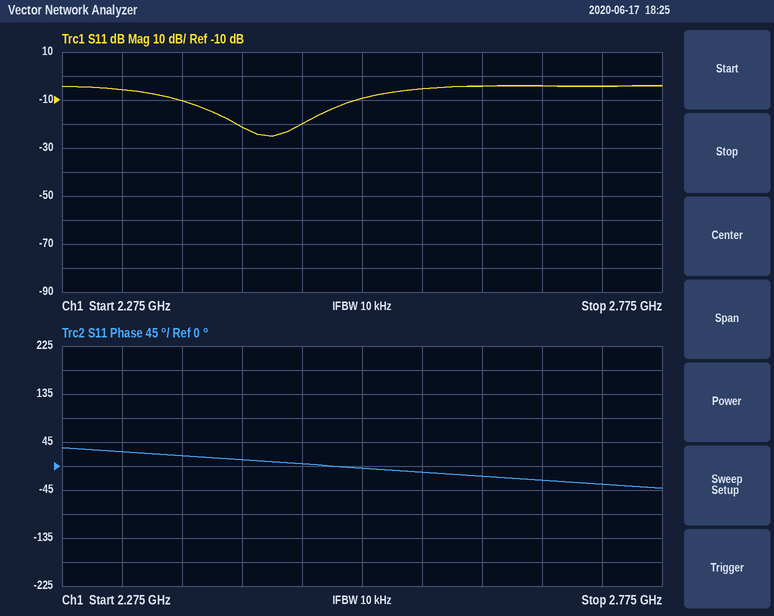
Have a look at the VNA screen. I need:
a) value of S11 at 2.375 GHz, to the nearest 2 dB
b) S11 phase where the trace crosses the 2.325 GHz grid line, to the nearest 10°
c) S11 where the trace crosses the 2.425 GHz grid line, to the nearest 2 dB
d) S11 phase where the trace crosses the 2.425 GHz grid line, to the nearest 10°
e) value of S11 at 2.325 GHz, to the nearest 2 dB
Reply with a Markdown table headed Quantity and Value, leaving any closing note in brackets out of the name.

| Quantity | Value |
|---|---|
| value of S11 at 2.375 GHz, to the nearest 2 dB | -10 dB |
| S11 phase where the trace crosses the 2.325 GHz grid line, to the nearest 10° | 30° |
| S11 where the trace crosses the 2.425 GHz grid line, to the nearest 2 dB | -22 dB |
| S11 phase where the trace crosses the 2.425 GHz grid line, to the nearest 10° | 10° |
| value of S11 at 2.325 GHz, to the nearest 2 dB | -6 dB |
